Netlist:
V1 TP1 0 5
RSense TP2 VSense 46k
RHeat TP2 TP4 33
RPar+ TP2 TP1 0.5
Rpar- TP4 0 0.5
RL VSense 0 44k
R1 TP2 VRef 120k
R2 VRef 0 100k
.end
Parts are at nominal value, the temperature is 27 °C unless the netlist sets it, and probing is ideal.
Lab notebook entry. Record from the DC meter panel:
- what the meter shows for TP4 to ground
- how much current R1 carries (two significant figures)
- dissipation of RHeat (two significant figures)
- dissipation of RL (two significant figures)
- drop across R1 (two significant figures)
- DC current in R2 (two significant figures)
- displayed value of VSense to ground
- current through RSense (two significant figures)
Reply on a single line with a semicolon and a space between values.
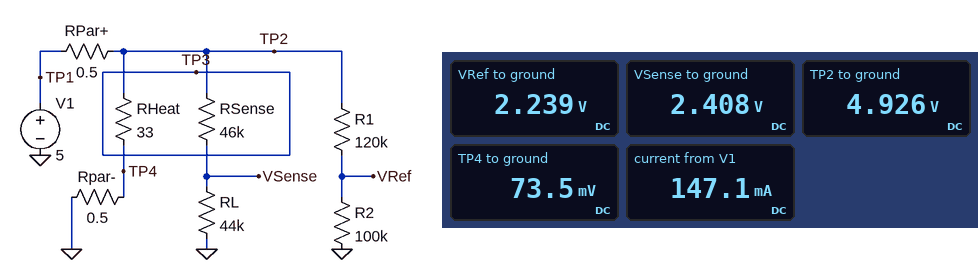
73.5 mV; 22 µA; 710 mW; 130 µW; 2.7 V; 22 µA; 2.408 V; 55 µA
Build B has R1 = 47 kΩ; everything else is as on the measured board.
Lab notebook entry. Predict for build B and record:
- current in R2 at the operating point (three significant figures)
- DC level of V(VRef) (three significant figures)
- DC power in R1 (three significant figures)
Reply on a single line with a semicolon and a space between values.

33.5 µA; 3.35 V; 52.8 µW
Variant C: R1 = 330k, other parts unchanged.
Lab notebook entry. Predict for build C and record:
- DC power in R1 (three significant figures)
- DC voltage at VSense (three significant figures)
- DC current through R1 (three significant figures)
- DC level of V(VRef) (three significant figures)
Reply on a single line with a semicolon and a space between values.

43.3 µW; 2.41 V; 11.5 µA; 1.15 V
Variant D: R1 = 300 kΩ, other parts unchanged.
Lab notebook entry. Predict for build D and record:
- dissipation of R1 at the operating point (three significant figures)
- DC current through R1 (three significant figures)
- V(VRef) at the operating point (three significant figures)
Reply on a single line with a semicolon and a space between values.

45.5 µW; 12.3 µA; 1.23 V
